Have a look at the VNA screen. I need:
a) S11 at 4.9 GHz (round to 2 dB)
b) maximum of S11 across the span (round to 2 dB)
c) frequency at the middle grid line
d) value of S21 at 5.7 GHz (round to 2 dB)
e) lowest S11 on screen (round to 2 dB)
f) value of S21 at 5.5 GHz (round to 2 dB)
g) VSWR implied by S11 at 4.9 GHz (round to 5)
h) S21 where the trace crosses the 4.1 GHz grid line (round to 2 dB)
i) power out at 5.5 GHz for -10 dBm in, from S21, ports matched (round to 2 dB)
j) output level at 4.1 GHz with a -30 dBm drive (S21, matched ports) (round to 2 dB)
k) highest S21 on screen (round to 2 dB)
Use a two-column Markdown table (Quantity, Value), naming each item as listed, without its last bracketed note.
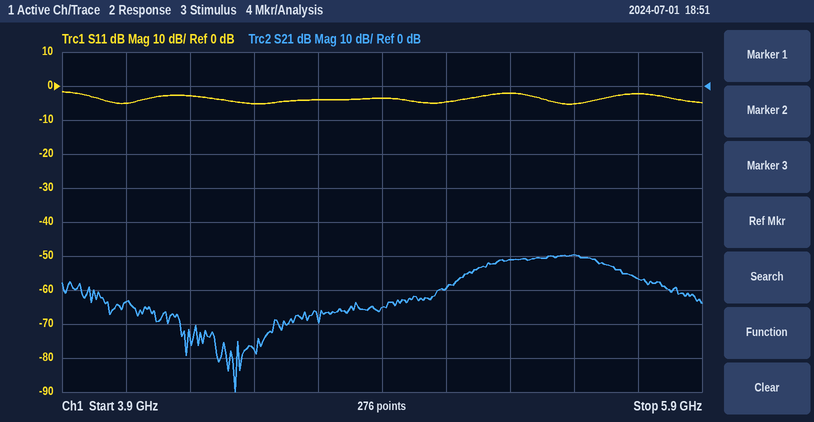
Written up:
| Quantity | Value |
|---|---|
| S11 at 4.9 GHz | -4 dB |
| maximum of S11 across the span | -2 dB |
| frequency at the middle grid line | 4.9 GHz |
| value of S21 at 5.7 GHz | -56 dB |
| lowest S11 on screen | -6 dB |
| value of S21 at 5.5 GHz | -50 dB |
| VSWR implied by S11 at 4.9 GHz | 5 |
| S21 where the trace crosses the 4.1 GHz grid line | -64 dB |
| power out at 5.5 GHz for -10 dBm in, from S21, ports matched | -60 dBm |
| output level at 4.1 GHz with a -30 dBm drive (S21, matched ports) | -94 dBm |
| highest S21 on screen | -50 dB |
